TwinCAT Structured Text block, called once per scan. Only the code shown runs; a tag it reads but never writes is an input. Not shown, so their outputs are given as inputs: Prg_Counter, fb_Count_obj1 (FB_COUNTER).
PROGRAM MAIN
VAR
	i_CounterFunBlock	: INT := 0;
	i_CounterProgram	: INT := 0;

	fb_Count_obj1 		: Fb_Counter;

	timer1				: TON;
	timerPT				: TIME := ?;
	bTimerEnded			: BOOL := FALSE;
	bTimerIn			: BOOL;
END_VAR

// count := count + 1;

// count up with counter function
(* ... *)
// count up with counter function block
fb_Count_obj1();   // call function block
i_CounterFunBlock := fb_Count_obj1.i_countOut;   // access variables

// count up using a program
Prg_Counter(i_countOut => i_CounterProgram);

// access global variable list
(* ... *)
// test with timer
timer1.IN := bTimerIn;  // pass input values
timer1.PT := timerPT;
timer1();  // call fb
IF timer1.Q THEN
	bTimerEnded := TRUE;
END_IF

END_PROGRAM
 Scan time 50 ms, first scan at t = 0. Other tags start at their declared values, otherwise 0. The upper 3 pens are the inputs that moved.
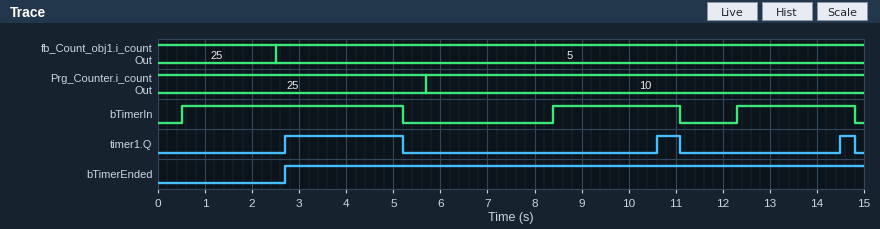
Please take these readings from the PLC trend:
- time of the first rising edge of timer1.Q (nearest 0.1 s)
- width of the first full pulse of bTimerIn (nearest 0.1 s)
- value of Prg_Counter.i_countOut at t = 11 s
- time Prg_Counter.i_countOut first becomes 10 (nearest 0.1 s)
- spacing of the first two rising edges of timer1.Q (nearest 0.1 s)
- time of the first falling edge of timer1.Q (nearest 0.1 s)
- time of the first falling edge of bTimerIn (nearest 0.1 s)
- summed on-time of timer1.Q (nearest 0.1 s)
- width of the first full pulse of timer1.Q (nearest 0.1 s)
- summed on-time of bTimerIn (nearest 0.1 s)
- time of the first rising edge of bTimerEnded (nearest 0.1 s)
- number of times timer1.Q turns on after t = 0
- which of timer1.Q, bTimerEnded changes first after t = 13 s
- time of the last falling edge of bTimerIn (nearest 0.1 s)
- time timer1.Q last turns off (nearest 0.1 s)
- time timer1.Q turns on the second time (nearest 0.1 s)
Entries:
2.7 s
4.7 s
10
5.7 s
7.9 s
5.2 s
5.2 s
3.3 s
2.5 s
9.9 s
2.7 s
3
timer1.Q
14.8 s
14.8 s
10.6 s
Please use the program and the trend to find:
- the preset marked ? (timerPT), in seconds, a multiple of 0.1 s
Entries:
2.2 s
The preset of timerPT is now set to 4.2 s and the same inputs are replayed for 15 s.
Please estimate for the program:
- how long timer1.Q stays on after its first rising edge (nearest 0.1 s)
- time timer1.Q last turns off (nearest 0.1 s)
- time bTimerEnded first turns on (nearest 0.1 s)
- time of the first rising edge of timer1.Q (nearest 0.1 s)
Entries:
0.5 s
5.2 s
4.7 s
4.7 s
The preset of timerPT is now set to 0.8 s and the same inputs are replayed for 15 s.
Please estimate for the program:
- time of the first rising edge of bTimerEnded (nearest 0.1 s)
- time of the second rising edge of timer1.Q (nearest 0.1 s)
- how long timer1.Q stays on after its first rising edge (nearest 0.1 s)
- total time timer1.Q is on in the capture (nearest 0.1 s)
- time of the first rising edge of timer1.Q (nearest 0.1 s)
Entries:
1.3 s
9.2 s
3.9 s
7.5 s
1.3 s
